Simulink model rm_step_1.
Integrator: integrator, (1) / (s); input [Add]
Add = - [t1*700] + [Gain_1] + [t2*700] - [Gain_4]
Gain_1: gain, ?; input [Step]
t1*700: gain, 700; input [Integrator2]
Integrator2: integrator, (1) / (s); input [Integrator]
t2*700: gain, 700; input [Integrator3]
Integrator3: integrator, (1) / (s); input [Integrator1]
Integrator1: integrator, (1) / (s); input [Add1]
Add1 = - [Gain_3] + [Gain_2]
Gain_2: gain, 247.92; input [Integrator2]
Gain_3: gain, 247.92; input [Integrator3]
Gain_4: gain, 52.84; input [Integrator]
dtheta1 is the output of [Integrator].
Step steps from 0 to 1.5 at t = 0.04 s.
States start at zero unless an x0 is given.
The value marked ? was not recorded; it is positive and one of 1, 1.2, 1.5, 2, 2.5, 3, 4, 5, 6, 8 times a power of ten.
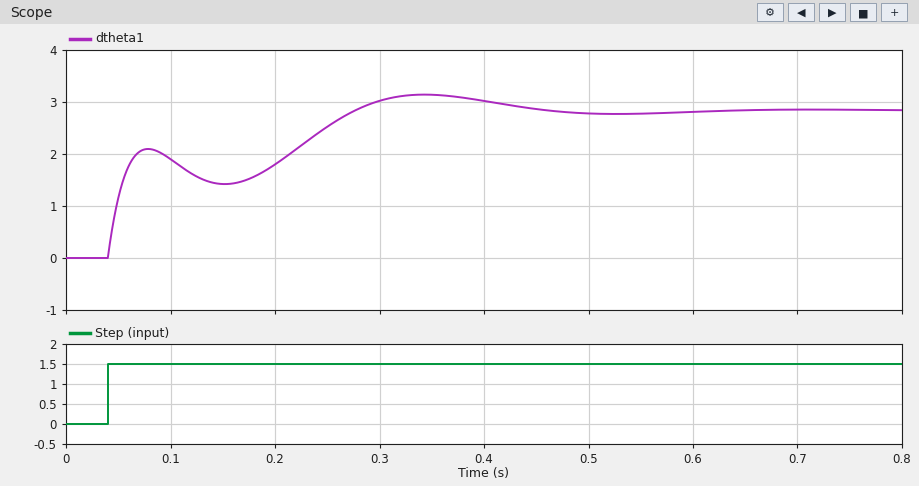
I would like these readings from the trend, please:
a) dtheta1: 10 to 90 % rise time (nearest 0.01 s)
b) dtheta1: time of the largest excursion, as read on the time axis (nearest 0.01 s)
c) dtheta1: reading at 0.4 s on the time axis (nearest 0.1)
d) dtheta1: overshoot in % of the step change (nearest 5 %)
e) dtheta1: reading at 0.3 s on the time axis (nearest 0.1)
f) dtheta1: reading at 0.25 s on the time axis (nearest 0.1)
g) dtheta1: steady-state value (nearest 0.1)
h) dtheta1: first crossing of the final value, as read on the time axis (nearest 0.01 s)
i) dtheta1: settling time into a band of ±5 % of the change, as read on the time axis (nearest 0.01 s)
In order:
0.21 s
0.34 s
3.0
10 %
3.0
2.5
2.8
0.28 s
0.41 s
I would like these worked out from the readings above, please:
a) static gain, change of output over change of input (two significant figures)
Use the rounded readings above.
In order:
1.9
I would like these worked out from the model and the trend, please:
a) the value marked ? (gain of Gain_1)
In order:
100
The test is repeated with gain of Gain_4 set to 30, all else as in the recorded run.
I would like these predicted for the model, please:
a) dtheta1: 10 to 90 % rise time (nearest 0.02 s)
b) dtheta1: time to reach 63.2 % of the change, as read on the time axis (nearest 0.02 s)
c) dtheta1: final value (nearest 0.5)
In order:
0.24 s
0.22 s
5.0
